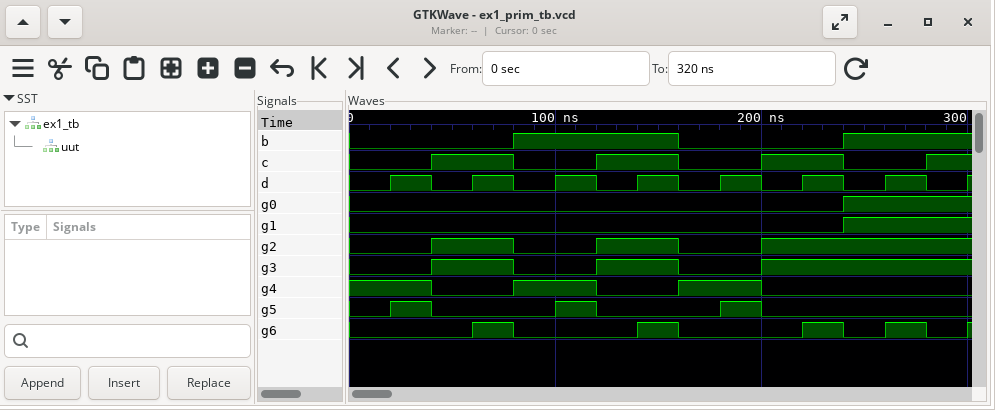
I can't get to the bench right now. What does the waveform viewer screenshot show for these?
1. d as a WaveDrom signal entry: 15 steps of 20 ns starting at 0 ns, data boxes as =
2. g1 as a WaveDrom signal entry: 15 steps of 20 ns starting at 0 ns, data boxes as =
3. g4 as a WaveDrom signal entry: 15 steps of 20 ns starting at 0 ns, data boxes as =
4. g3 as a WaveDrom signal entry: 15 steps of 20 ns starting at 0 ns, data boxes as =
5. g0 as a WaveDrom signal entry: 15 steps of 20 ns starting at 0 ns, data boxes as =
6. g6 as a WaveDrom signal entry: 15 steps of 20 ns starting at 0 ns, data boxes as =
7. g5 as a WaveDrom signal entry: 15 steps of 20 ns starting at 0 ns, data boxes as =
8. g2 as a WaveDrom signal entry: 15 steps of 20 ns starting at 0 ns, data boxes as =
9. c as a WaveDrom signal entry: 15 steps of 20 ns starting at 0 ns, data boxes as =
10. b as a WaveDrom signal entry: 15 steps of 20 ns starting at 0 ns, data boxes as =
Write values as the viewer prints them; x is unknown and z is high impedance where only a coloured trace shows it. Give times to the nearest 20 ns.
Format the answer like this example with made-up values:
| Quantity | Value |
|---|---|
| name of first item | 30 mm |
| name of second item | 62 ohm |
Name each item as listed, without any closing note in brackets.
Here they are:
| Quantity | Value |
|---|---|
| d as a WaveDrom signal entry: 15 steps of 20 ns starting at 0 ns, data boxes as = | {name: 'd', wave: '010101010101010'} |
| g1 as a WaveDrom signal entry: 15 steps of 20 ns starting at 0 ns, data boxes as = | {name: 'g1', wave: '0...........1..'} |
| g4 as a WaveDrom signal entry: 15 steps of 20 ns starting at 0 ns, data boxes as = | {name: 'g4', wave: '1.0.1.0.1.0....'} |
| g3 as a WaveDrom signal entry: 15 steps of 20 ns starting at 0 ns, data boxes as = | {name: 'g3', wave: '0.1.0.1.0.1....'} |
| g0 as a WaveDrom signal entry: 15 steps of 20 ns starting at 0 ns, data boxes as = | {name: 'g0', wave: '0...........1..'} |
| g6 as a WaveDrom signal entry: 15 steps of 20 ns starting at 0 ns, data boxes as = | {name: 'g6', wave: '0..10..10..1010'} |
| g5 as a WaveDrom signal entry: 15 steps of 20 ns starting at 0 ns, data boxes as = | {name: 'g5', wave: '010..10..10....'} |
| g2 as a WaveDrom signal entry: 15 steps of 20 ns starting at 0 ns, data boxes as = | {name: 'g2', wave: '0.1.0.1.0.1....'} |
| c as a WaveDrom signal entry: 15 steps of 20 ns starting at 0 ns, data boxes as = | {name: 'c', wave: '0.1.0.1.0.1.0.1'} |
| b as a WaveDrom signal entry: 15 steps of 20 ns starting at 0 ns, data boxes as = | {name: 'b', wave: '0...1...0...1..'} |
